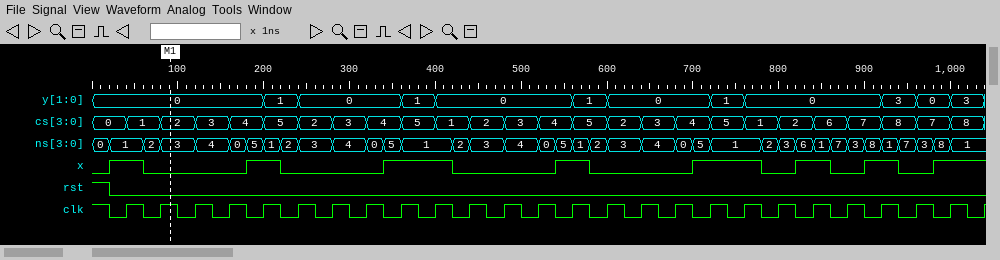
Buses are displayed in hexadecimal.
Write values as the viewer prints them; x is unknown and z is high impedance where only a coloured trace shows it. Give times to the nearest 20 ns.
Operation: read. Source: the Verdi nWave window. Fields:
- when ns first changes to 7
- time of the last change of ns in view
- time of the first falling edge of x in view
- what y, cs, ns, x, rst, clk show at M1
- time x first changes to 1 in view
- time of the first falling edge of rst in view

860 ns
1000 ns
60 ns
y=0, cs=2, ns=3, x=0, rst=0, clk=1
20 ns
20 ns
